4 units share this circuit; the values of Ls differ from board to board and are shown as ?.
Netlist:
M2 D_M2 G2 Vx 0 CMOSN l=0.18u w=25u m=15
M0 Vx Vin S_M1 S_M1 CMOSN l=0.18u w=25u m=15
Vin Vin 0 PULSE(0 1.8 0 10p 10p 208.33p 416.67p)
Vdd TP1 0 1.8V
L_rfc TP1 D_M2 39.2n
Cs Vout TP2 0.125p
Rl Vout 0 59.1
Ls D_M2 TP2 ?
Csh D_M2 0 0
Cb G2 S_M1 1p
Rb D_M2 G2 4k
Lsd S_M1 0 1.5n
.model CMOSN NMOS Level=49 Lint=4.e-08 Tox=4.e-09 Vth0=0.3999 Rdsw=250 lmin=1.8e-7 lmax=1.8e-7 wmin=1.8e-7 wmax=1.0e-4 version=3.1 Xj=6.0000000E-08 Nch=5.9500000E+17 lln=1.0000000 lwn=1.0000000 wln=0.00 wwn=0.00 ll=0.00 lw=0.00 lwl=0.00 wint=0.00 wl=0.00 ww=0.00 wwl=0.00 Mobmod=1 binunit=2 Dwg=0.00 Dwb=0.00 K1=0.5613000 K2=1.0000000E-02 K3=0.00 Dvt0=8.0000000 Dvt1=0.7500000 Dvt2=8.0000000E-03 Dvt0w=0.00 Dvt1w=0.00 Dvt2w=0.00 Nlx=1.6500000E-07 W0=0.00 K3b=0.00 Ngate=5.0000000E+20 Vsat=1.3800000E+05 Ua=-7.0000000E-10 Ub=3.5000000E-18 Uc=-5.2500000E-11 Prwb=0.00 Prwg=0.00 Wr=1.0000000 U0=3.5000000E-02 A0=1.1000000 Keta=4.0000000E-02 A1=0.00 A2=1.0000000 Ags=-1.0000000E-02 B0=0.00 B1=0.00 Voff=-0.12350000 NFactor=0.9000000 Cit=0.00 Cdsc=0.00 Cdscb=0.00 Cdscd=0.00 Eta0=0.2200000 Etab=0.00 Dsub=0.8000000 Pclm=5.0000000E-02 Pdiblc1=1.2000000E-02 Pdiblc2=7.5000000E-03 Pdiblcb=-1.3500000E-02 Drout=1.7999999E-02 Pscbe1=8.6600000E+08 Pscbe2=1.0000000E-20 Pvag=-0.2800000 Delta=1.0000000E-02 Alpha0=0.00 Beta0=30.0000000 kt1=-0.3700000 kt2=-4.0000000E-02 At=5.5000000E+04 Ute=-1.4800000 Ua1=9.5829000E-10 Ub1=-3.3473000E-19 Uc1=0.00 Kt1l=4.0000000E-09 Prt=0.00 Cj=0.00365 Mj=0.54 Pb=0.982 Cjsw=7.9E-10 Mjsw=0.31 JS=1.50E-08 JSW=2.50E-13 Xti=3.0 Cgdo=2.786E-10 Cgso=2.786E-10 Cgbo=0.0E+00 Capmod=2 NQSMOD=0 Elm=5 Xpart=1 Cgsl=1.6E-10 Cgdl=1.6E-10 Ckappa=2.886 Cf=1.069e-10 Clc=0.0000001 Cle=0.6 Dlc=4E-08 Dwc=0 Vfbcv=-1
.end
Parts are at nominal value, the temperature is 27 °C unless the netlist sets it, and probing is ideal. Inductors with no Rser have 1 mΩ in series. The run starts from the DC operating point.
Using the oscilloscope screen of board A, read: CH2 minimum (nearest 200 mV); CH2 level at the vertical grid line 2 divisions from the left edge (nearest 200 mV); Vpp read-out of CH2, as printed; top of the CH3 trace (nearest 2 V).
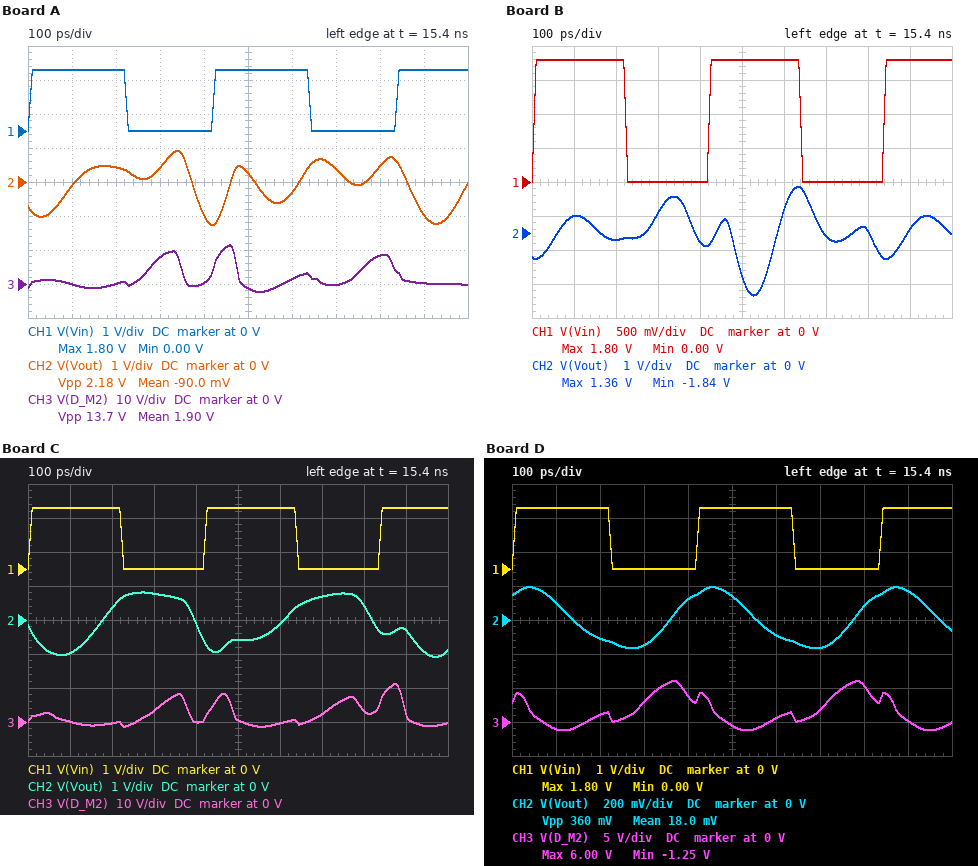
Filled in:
-1.2 V
400 mV
2.18 V
12 V
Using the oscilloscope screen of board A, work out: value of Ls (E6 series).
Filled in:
15 nH
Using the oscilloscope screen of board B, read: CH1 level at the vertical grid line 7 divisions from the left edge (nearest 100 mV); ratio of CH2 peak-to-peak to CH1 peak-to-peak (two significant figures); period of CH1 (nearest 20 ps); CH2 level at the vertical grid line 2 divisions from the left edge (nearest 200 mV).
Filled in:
0 V
1.8
420 ps
-200 mV
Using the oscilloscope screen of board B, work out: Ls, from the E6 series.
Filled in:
10 nH
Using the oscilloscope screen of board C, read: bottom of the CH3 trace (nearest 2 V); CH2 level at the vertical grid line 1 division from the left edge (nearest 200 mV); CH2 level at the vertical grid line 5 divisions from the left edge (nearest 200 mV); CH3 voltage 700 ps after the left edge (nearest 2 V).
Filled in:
-2 V
-1.0 V
-600 mV
2 V
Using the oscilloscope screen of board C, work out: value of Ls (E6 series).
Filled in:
22 nH
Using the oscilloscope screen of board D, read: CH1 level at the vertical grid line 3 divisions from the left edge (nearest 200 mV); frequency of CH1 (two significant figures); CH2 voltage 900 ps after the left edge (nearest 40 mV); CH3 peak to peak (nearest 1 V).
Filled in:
0 V
2.4 GHz
160 mV
7 V
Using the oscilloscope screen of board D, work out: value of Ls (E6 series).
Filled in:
100 nH
